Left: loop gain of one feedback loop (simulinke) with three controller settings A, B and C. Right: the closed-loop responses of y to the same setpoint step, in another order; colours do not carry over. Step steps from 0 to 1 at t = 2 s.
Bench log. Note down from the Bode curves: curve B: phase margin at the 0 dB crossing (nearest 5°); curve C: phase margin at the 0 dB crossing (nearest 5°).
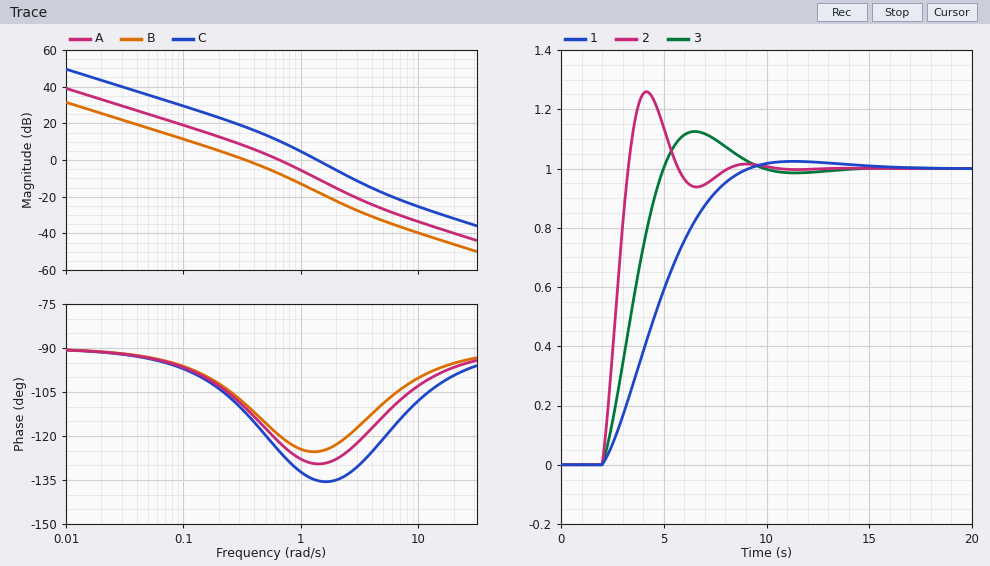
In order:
70°
45°
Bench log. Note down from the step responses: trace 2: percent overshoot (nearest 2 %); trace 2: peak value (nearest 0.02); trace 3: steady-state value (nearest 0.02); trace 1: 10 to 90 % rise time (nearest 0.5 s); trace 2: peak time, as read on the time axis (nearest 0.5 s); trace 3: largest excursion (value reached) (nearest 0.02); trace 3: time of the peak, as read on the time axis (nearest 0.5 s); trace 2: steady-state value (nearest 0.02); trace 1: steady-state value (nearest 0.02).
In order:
26 %
1.26
1.00
4.5 s
4.0 s
1.12
6.5 s
1.00
1.00
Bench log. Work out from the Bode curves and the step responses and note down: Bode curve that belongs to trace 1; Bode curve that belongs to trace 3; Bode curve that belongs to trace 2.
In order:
B
A
C
